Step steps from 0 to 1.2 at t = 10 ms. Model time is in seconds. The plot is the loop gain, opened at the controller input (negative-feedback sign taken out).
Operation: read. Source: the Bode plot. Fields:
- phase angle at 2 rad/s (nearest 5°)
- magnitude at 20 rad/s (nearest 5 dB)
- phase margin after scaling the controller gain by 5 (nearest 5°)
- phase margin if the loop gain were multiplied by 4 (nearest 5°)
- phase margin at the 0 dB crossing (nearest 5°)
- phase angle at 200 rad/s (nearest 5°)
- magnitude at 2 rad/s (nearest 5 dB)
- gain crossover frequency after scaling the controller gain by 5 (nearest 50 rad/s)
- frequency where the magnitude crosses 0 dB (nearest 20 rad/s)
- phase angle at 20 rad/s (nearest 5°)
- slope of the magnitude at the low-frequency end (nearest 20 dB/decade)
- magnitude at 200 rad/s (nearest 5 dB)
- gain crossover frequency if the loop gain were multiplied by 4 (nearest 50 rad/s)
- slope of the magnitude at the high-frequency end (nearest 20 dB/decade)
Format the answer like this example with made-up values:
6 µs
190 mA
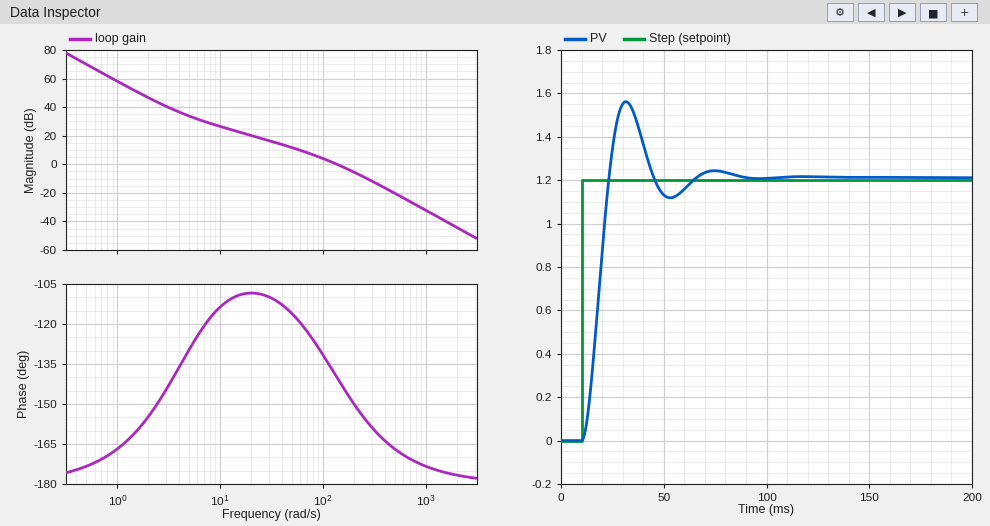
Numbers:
-155°
20 dB
20°
20°
40°
-150°
45 dB
350 rad/s
140 rad/s
-110°
-40 dB/decade
-5 dB
300 rad/s
-40 dB/decade
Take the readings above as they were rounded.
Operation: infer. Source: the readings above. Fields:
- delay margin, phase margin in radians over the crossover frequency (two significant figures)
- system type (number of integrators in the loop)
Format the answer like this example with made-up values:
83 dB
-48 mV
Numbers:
0.0050 s
2
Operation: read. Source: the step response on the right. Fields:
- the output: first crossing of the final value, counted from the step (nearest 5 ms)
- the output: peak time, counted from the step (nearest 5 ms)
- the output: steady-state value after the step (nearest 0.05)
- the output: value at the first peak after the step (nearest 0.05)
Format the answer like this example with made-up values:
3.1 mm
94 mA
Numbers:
15 ms
20 ms
1.20
1.55
